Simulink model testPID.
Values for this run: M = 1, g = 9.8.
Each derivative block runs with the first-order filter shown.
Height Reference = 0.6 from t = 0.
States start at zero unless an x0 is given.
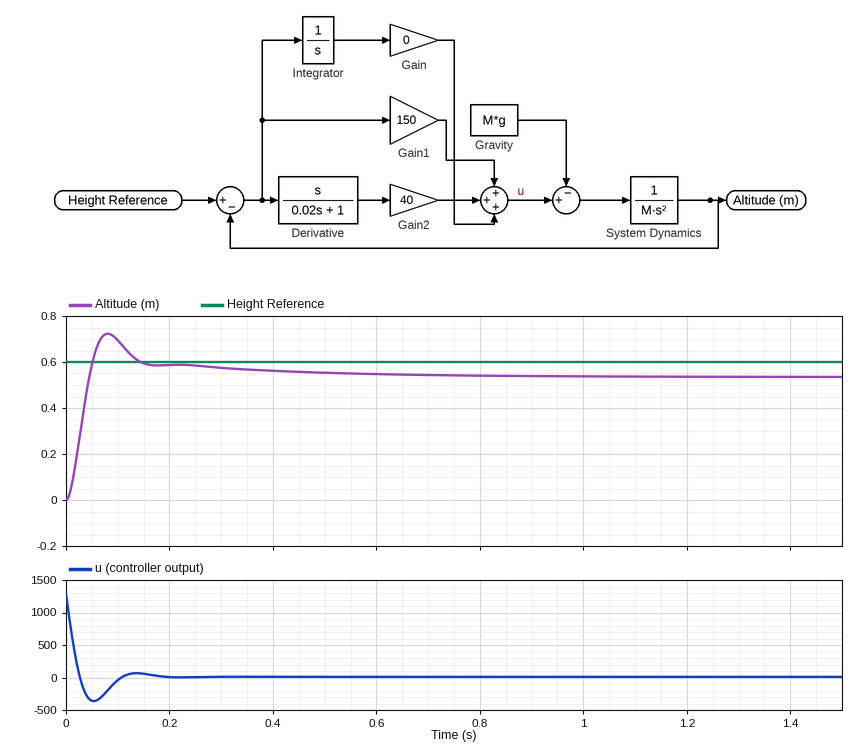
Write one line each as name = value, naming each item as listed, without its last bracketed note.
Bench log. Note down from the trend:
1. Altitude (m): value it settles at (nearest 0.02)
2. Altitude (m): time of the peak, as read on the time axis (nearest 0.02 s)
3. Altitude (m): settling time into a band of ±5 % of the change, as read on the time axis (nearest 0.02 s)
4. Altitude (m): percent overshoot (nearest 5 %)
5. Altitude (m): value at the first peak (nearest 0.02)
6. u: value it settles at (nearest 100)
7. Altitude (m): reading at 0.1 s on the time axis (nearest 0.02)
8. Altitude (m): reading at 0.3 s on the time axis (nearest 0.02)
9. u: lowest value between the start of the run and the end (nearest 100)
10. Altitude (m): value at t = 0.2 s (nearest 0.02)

Altitude (m): value it settles at = 0.54
Altitude (m): time of the peak, as read on the time axis = 0.08 s
Altitude (m): settling time into a band of ±5 % of the change, as read on the time axis = 0.40 s
Altitude (m): percent overshoot = 35 %
Altitude (m): value at the first peak = 0.72
u: value it settles at = 0
Altitude (m): reading at 0.1 s on the time axis = 0.70
Altitude (m): reading at 0.3 s on the time axis = 0.58
u: lowest value between the start of the run and the end = -400
Altitude (m): value at t = 0.2 s = 0.58
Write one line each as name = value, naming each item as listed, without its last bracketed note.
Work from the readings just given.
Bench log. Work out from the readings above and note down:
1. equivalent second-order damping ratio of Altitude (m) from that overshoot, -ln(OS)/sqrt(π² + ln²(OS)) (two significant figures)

equivalent second-order damping ratio of Altitude (m) from that overshoot, -ln(OS)/sqrt(π² + ln²(OS)) = 0.32
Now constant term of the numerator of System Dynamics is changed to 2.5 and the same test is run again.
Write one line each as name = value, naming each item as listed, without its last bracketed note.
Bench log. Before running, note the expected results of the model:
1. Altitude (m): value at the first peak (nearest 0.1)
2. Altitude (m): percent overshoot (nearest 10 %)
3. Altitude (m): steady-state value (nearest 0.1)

Altitude (m): value at the first peak = 0.8
Altitude (m): percent overshoot = 50 %
Altitude (m): steady-state value = 0.5
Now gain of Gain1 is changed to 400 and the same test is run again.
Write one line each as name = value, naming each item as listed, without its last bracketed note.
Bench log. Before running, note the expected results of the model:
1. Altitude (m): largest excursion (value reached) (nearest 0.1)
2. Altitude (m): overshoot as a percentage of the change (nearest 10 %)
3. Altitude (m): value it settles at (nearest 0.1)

Altitude (m): largest excursion (value reached) = 0.8
Altitude (m): overshoot as a percentage of the change = 40 %
Altitude (m): value it settles at = 0.6
